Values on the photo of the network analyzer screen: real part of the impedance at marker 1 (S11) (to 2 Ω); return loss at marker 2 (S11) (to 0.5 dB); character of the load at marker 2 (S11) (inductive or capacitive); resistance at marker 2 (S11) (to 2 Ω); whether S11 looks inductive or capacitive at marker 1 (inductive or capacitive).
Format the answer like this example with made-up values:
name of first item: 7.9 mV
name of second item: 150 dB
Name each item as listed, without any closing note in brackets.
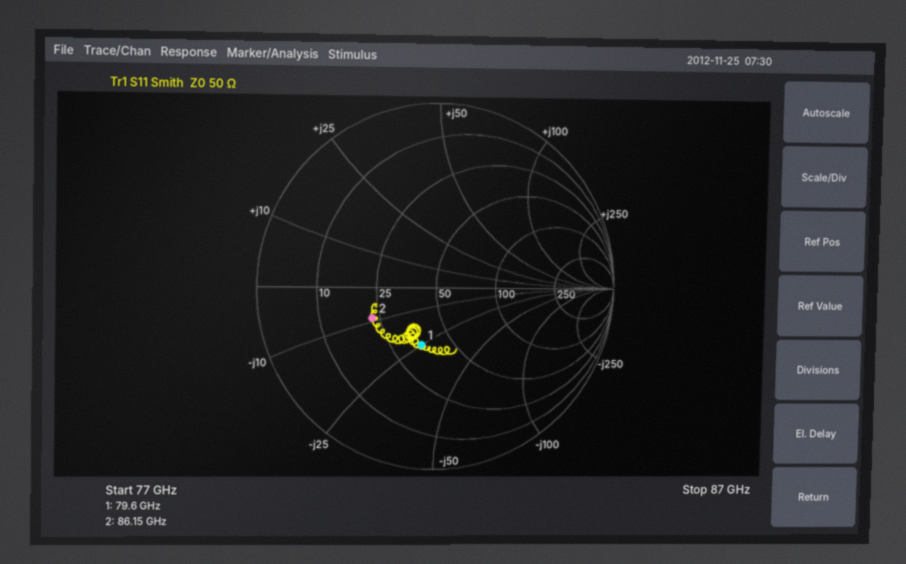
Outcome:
real part of the impedance at marker 1 (S11): 36 Ω
return loss at marker 2 (S11): 8.0 dB
character of the load at marker 2 (S11): capacitive
resistance at marker 2 (S11): 22 Ω
whether S11 looks inductive or capacitive at marker 1: capacitive
